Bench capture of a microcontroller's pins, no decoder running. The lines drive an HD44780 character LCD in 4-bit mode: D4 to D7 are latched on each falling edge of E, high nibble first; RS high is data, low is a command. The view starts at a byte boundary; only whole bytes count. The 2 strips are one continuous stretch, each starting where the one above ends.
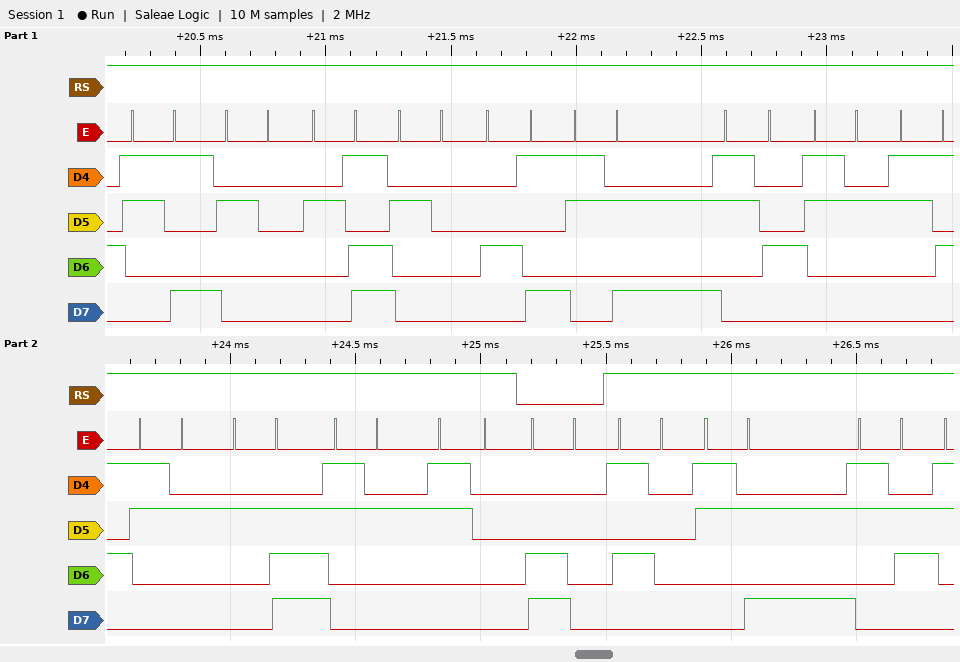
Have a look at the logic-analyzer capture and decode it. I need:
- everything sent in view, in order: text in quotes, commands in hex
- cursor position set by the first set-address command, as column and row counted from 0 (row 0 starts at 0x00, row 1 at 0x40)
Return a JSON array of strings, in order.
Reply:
["\"9 - I:4252.20\" 0xC0 \"P:6\"", "column 0, row 1"]
